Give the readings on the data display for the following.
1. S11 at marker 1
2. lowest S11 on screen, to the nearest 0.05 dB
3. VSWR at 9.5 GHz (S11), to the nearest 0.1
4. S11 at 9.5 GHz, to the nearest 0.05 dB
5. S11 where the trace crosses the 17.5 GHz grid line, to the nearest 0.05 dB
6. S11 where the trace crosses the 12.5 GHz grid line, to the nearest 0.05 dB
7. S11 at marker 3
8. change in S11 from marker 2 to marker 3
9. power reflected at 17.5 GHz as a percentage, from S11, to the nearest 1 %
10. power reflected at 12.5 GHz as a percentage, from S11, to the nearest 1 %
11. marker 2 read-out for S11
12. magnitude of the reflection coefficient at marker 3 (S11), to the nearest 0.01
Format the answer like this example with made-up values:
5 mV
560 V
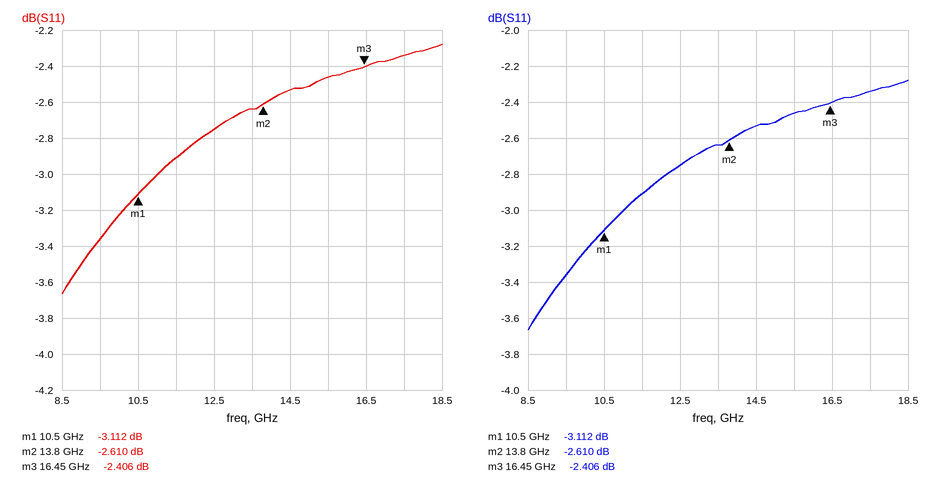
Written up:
-3.112 dB
-3.65 dB
5.2
-3.35 dB
-2.35 dB
-2.75 dB
-2.406 dB
0.204 dB
58 %
53 %
-2.610 dB
0.76
